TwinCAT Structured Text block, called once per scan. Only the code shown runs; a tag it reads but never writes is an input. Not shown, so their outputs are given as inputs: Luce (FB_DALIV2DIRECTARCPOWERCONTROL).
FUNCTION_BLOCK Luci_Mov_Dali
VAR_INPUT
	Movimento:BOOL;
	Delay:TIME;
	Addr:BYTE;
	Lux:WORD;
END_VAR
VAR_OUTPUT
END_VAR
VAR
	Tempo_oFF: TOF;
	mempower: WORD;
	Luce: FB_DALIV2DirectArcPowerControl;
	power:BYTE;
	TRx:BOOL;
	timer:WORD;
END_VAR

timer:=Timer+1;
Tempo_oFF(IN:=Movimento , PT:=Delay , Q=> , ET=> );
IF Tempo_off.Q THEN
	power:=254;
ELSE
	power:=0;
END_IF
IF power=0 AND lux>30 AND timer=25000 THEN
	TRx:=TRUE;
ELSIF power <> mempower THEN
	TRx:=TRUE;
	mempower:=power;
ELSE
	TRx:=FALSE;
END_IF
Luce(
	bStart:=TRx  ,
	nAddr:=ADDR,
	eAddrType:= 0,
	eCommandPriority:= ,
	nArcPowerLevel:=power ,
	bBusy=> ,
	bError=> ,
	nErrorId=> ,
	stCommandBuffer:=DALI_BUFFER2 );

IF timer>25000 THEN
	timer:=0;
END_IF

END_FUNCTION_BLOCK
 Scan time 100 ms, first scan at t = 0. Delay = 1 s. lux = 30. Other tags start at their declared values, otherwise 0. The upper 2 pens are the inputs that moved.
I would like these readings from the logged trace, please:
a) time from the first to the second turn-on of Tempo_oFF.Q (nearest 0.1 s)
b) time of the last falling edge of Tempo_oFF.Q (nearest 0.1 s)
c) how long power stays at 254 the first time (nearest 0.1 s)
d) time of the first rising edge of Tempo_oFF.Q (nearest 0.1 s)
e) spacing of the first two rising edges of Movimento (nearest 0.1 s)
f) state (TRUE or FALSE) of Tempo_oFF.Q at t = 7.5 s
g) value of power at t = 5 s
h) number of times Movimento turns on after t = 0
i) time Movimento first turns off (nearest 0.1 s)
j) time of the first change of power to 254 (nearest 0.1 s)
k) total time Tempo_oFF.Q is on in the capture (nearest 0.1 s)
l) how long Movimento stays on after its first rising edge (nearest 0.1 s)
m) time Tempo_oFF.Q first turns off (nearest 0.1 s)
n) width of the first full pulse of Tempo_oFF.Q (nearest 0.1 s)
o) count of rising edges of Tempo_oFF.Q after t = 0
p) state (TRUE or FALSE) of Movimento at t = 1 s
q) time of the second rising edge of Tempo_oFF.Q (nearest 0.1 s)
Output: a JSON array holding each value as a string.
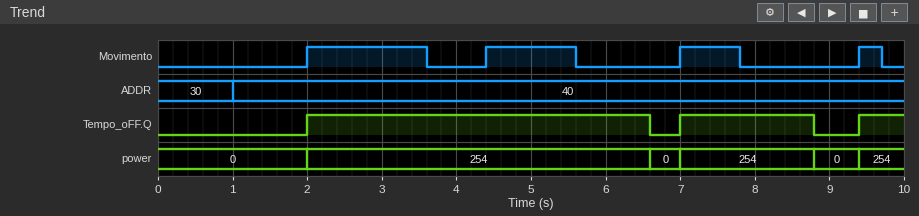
["5.0 s", "8.8 s", "4.6 s", "2.0 s", "2.4 s", "TRUE", "254", "4", "3.6 s", "2.0 s", "7.0 s", "1.6 s", "6.6 s", "4.6 s", "3", "FALSE", "7.0 s"]
